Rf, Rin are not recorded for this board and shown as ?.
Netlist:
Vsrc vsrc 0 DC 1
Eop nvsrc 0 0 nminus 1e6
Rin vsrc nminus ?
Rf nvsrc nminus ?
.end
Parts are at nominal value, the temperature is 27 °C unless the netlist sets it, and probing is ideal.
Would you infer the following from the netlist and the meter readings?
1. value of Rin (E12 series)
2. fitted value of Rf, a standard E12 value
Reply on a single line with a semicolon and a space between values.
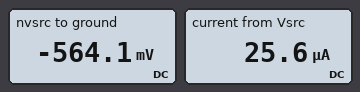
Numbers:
39 kΩ; 22 kΩ
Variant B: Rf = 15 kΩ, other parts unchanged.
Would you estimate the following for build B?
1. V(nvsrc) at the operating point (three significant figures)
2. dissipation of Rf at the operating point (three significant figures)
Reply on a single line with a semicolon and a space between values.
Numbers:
-385 mV; 9.86 µW
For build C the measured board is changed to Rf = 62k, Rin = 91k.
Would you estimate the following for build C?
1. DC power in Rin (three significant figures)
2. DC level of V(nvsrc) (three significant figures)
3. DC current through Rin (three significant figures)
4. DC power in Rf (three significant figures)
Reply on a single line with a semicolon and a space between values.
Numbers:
11.0 µW; -681 mV; 11.0 µA; 7.49 µW
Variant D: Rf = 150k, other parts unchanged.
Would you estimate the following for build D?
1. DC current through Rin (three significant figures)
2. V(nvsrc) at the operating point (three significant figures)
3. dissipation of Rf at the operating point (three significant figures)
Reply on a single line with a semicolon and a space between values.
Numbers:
25.6 µA; -3.85 V; 98.6 µW
